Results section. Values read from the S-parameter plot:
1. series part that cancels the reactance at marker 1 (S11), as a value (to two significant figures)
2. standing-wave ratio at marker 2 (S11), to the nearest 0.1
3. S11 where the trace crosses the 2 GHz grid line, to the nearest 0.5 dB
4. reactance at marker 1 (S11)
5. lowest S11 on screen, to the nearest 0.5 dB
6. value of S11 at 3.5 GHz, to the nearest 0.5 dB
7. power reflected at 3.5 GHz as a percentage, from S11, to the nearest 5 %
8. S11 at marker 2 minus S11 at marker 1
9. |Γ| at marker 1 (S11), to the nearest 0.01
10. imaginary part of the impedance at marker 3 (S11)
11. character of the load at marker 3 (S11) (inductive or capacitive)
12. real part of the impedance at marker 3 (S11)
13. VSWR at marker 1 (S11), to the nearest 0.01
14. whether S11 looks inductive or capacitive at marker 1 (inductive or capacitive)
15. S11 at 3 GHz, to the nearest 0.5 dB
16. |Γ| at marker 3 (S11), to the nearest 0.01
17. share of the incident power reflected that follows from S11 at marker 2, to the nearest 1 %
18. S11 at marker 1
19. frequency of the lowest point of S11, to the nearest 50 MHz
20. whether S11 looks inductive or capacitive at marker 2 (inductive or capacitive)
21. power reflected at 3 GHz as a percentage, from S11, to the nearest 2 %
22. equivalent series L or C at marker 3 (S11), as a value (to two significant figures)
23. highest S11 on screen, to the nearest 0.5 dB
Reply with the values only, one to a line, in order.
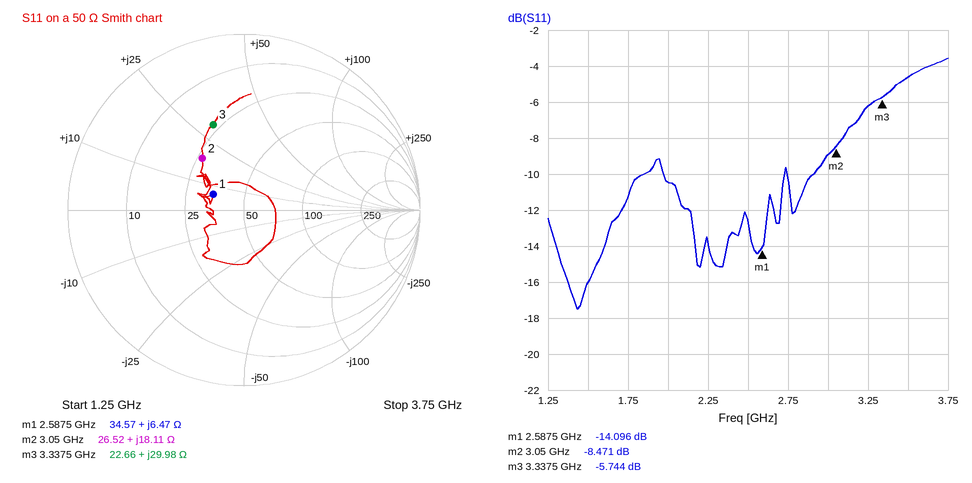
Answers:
9.5 pF
2.2
-10.5 dB
+6.47 Ω
-17.5 dB
-4.5 dB
35 %
5.625 dB
0.20
+29.98 Ω
inductive
22.66 Ω
1.49
inductive
-9.0 dB
0.52
14 %
-14.096 dB
1.45 GHz
inductive
12 %
1.4 nH
-3.5 dB
